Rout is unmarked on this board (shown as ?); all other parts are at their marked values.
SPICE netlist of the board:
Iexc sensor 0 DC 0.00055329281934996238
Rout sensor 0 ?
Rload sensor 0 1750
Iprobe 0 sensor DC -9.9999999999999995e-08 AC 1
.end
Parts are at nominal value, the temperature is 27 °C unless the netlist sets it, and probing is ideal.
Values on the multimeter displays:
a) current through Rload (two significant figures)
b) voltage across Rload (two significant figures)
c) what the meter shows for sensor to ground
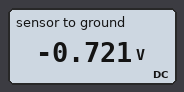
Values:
410 µA
720 mV
-0.721 V
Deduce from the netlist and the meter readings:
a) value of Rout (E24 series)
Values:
5.1 kΩ
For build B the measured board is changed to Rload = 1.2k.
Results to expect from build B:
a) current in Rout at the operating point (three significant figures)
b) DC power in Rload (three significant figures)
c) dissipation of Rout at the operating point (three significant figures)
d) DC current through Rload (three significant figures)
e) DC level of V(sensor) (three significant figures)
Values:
105 µA
241 µW
56.7 µW
448 µA
-538 mV
